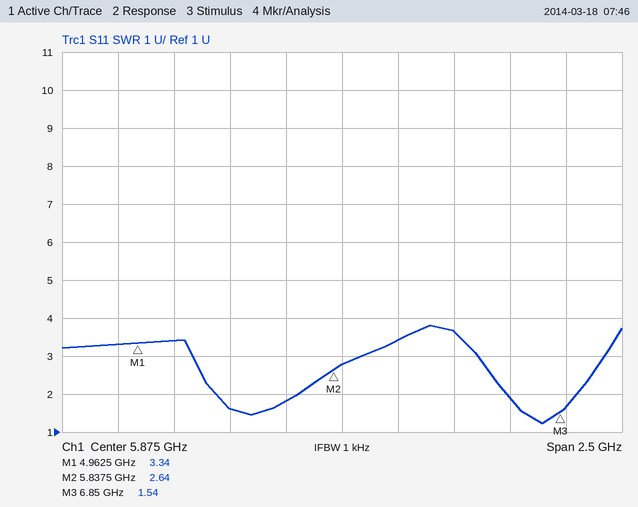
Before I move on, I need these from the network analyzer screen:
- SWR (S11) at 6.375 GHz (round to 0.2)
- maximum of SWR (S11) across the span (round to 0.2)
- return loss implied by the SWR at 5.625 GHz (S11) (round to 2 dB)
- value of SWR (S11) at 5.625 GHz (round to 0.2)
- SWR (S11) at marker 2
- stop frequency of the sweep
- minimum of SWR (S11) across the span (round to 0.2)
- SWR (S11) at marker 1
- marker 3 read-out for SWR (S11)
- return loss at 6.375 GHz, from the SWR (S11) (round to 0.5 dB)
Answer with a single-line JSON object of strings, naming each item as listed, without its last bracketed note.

{"SWR (S11) at 6.375 GHz": "3.6", "maximum of SWR (S11) across the span": "3.8", "return loss implied by the SWR at 5.625 GHz (S11)": "10 dB", "value of SWR (S11) at 5.625 GHz": "1.8", "SWR (S11) at marker 2": "2.64", "stop frequency of the sweep": "7.125 GHz", "minimum of SWR (S11) across the span": "1.2", "SWR (S11) at marker 1": "3.34", "marker 3 read-out for SWR": "1.54", "return loss at 6.375 GHz, from the SWR (S11)": "5.0 dB"}
